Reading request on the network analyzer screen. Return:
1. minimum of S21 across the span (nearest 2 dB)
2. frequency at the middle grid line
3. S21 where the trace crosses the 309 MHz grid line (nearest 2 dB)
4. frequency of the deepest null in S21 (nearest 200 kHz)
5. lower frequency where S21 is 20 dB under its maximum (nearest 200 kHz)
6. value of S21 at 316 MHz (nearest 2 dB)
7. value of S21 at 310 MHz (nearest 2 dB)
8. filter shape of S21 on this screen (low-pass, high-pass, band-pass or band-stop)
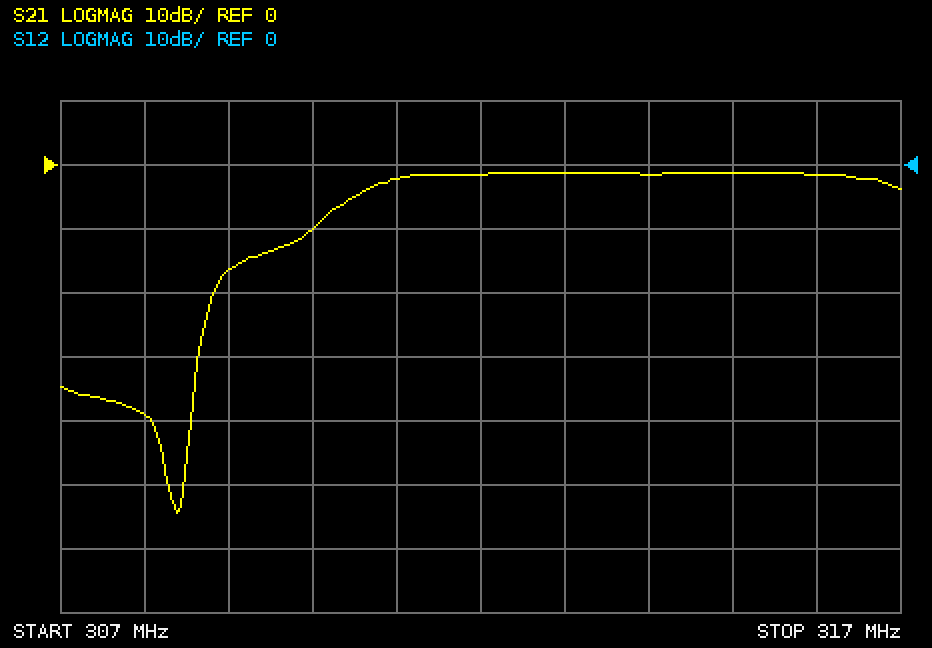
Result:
-54 dB
312 MHz
-16 dB
308.4 MHz
308.8 MHz
-2 dB
-10 dB
high-pass
